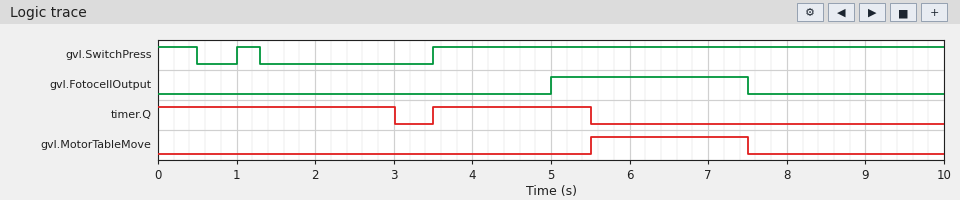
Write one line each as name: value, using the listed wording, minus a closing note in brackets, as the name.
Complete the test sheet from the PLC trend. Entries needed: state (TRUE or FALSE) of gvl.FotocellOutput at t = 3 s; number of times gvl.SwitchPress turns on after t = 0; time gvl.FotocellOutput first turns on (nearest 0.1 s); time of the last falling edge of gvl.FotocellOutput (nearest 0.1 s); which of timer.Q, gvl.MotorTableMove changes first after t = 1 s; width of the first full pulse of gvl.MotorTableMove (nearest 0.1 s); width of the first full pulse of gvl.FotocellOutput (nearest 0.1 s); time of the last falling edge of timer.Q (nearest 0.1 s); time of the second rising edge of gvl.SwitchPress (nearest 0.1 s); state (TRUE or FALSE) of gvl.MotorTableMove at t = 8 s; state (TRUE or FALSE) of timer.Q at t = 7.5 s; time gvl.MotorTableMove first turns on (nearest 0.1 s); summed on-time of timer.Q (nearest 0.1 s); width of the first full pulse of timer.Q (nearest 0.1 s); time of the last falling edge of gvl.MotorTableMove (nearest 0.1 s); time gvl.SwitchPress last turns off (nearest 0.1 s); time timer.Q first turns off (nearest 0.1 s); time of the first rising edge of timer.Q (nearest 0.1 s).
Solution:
state (TRUE or FALSE) of gvl.FotocellOutput at t = 3 s: FALSE
number of times gvl.SwitchPress turns on after t = 0: 2
time gvl.FotocellOutput first turns on: 5.0 s
time of the last falling edge of gvl.FotocellOutput: 7.5 s
which of timer.Q, gvl.MotorTableMove changes first after t = 1 s: timer.Q
width of the first full pulse of gvl.MotorTableMove: 2.0 s
width of the first full pulse of gvl.FotocellOutput: 2.5 s
time of the last falling edge of timer.Q: 5.5 s
time of the second rising edge of gvl.SwitchPress: 3.5 s
state (TRUE or FALSE) of gvl.MotorTableMove at t = 8 s: FALSE
state (TRUE or FALSE) of timer.Q at t = 7.5 s: FALSE
time gvl.MotorTableMove first turns on: 5.5 s
summed on-time of timer.Q: 5.0 s
width of the first full pulse of timer.Q: 2.0 s
time of the last falling edge of gvl.MotorTableMove: 7.5 s
time gvl.SwitchPress last turns off: 1.3 s
time timer.Q first turns off: 3.0 s
time of the first rising edge of timer.Q: 3.5 s
